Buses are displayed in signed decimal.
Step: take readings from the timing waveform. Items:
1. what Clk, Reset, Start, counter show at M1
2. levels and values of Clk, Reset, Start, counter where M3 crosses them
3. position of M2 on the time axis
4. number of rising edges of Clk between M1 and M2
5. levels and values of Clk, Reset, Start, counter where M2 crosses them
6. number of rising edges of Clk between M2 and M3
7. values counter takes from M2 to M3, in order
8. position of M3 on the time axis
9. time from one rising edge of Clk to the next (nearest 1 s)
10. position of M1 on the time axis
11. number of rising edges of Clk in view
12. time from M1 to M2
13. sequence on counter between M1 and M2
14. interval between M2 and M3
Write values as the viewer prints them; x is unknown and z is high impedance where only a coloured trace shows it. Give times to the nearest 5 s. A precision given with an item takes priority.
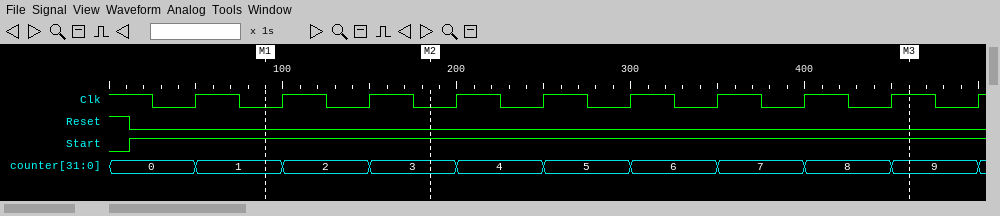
Clk=0, Reset=0, Start=1, counter=1
Clk=1, Reset=0, Start=1, counter=9
185 s
2
Clk=0, Reset=0, Start=1, counter=3
6
3, 4, 5, 6, 7, 8, 9
460 s
50 s
90 s
10
95 s
1, 2, 3
275 s
